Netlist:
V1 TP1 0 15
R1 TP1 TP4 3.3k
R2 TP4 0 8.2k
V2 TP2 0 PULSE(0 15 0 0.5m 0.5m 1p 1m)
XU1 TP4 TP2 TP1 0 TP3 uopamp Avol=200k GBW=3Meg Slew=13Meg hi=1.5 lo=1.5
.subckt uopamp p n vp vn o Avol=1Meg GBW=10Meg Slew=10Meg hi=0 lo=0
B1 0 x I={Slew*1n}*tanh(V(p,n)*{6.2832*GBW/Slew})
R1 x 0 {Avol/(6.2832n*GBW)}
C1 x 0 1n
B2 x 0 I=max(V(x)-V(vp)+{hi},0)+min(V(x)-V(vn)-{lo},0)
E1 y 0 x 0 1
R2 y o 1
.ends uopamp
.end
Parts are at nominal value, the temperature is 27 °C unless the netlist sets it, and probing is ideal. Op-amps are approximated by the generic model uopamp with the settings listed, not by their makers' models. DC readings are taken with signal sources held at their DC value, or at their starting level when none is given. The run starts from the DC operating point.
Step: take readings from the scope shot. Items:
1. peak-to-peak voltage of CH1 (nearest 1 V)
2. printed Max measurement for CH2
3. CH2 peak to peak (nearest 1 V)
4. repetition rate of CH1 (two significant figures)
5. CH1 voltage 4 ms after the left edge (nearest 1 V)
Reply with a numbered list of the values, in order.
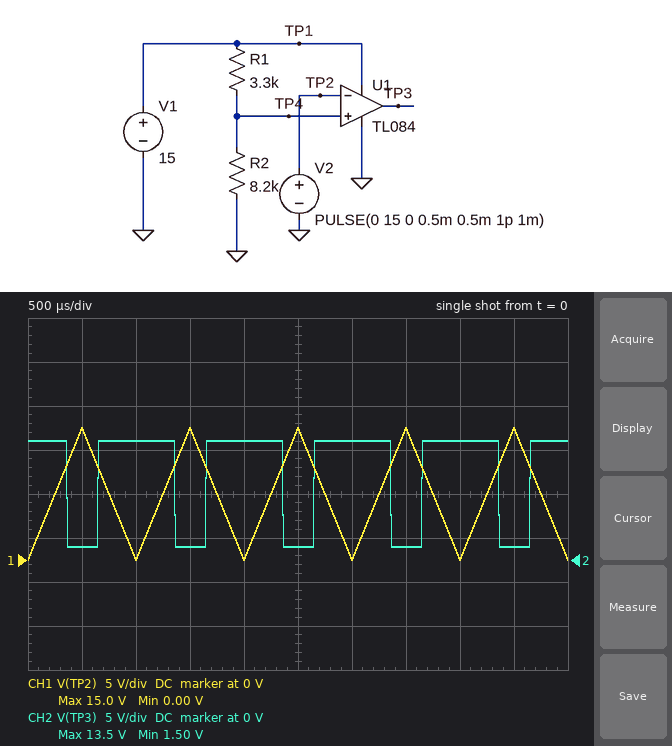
1. 15 V
2. 13.5 V
3. 12 V
4. 1.0 kHz
5. 0 V
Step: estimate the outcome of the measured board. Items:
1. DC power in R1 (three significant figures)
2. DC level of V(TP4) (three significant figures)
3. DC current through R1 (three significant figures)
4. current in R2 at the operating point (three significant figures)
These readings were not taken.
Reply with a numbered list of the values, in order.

1. 5.61 mW
2. 10.7 V
3. 1.30 mA
4. 1.30 mA
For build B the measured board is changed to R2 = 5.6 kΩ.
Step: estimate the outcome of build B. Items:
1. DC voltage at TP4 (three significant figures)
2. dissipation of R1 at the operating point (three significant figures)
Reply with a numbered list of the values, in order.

1. 9.44 V
2. 9.37 mW
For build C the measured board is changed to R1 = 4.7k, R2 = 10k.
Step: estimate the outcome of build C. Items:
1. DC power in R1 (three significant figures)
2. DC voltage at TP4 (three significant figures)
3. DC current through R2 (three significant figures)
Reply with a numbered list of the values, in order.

1. 4.89 mW
2. 10.2 V
3. 1.02 mA
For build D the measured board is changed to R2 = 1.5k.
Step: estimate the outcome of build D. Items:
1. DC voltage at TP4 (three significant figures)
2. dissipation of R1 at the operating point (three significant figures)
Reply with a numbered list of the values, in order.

1. 4.69 V
2. 32.2 mW
